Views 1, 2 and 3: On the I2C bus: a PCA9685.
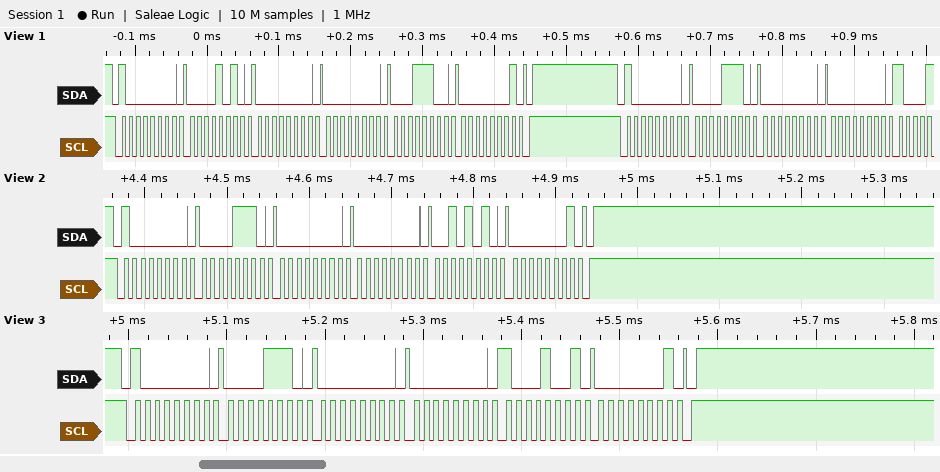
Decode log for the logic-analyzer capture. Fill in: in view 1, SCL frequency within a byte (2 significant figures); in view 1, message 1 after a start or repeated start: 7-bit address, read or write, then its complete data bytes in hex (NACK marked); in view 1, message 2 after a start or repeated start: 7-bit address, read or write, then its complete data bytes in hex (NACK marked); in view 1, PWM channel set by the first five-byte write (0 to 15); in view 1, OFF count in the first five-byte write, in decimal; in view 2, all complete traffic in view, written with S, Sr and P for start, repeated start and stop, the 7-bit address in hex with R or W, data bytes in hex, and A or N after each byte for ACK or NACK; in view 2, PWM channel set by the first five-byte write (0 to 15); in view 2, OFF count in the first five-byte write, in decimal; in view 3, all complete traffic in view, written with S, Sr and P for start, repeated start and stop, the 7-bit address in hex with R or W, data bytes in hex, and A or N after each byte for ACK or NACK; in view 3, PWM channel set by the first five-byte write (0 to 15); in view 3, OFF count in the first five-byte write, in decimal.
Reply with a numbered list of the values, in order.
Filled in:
1. 100 kHz
2. 0x40 write: 0A 00 00 1C 01
3. 0x40 write: 0E 00 00
4. 1
5. 284
6. S 40W A 0E A 00 A 00 A 2A A 01 A P
7. 2
8. 298
9. S 40W A 0E A 00 A 00 A 89 A 01 A P
10. 2
11. 393
